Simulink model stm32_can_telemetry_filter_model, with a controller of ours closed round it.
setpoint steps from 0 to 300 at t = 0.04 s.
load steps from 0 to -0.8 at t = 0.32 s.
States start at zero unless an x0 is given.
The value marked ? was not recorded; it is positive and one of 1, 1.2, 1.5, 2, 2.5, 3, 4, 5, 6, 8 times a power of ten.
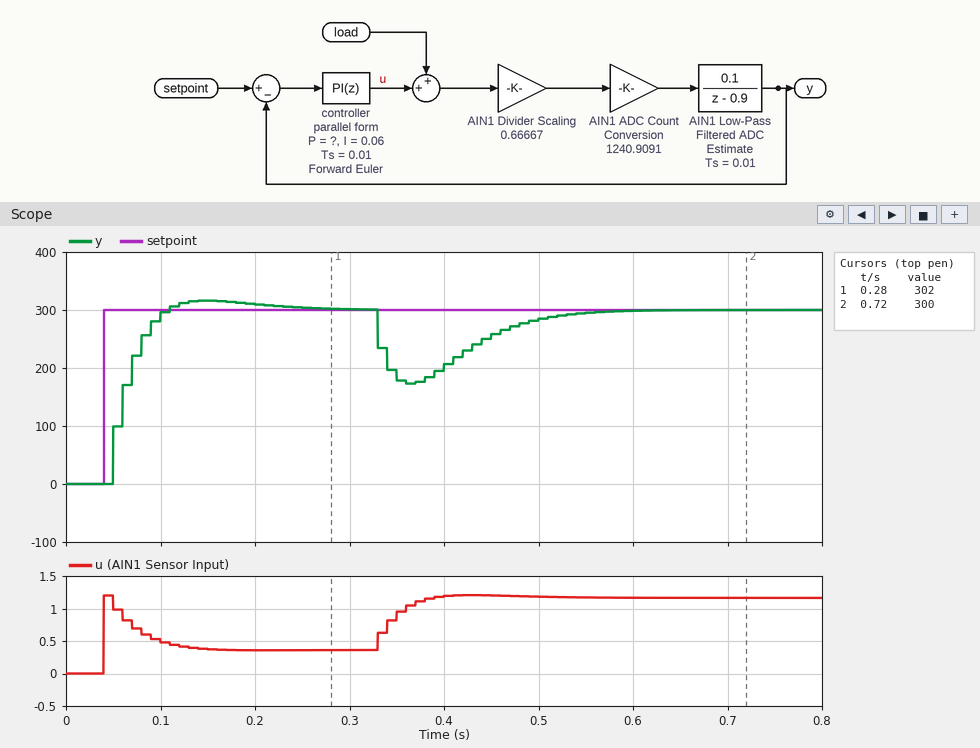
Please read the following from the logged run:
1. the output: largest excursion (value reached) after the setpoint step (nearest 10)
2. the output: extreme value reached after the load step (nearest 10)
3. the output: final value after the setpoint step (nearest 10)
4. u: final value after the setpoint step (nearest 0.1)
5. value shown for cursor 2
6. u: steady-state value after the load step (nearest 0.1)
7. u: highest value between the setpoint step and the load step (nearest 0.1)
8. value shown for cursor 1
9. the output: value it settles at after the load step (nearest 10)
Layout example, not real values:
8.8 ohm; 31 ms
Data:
320; 170; 300; 0.4; 300; 1.2; 1.2; 302; 300
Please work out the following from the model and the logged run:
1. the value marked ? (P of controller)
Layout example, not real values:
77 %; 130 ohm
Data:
0.004
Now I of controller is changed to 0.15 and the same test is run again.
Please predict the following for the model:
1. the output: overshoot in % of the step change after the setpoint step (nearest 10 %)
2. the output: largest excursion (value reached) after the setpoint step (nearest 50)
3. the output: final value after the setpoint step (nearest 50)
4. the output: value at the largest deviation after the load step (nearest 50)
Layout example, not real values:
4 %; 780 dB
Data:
30 %; 400; 300; 200
